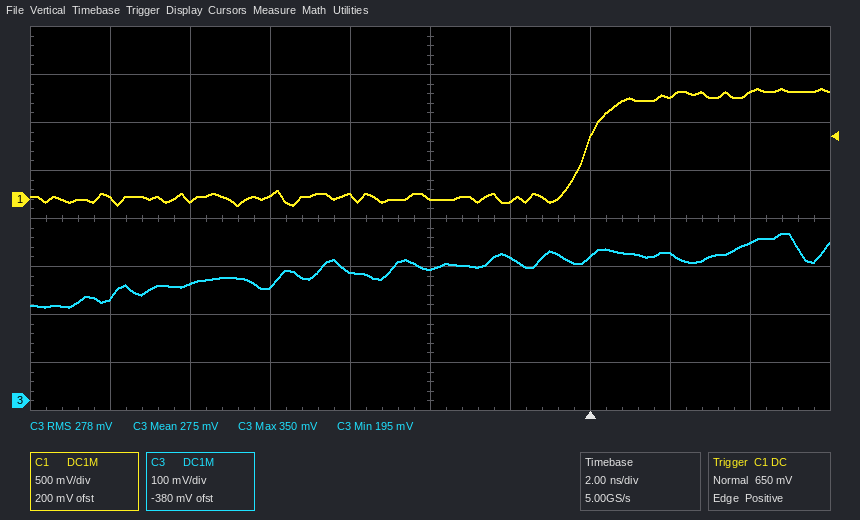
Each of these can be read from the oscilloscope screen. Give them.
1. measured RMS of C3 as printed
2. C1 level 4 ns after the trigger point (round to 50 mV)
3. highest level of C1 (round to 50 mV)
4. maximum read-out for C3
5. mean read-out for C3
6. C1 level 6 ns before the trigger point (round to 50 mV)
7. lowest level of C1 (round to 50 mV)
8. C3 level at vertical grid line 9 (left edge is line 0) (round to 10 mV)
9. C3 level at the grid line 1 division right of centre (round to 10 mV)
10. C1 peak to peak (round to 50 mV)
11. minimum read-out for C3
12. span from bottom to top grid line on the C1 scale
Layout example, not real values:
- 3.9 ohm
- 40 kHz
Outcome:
- 278 mV
- 1.10 V
- 1.15 V
- 350 mV
- 275 mV
- 50 mV
- -50 mV
- 330 mV
- 300 mV
- 1.20 V
- 195 mV
- 4 V
